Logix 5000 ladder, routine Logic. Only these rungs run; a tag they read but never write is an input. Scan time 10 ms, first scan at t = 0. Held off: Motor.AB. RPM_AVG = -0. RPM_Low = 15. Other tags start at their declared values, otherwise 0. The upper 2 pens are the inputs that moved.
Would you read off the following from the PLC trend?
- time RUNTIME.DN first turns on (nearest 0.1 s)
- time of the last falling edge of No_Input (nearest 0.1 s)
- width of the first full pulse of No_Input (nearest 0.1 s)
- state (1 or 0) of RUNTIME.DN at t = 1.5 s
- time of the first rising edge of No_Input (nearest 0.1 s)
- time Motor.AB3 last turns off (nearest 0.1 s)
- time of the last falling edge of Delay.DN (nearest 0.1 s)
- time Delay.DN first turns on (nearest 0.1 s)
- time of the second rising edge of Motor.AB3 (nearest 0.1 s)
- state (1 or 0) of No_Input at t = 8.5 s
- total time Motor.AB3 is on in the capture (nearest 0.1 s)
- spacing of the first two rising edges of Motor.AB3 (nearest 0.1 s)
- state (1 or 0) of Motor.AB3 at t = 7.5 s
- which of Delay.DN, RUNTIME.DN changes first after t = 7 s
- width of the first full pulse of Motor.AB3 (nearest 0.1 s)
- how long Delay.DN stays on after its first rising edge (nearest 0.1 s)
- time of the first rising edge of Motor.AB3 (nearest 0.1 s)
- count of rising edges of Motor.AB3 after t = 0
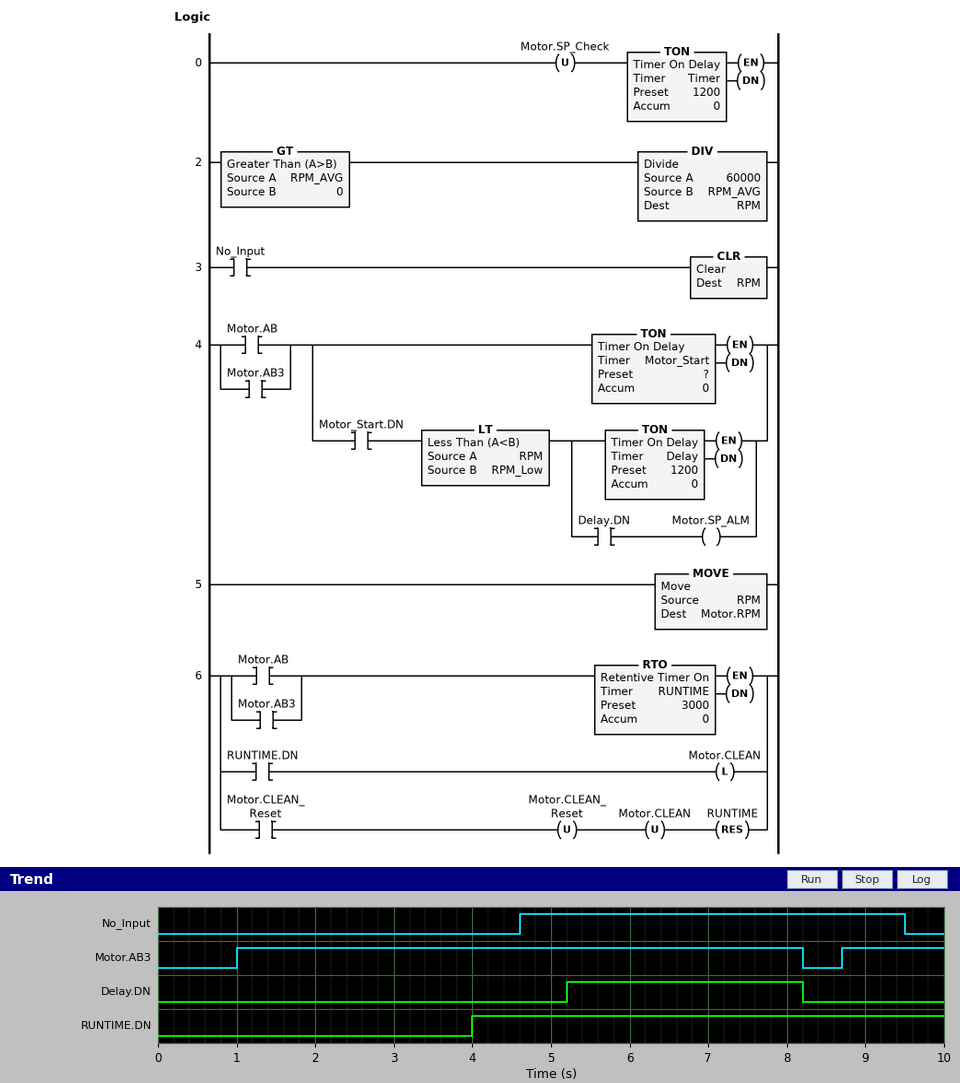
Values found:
4.0 s
9.5 s
4.9 s
0
4.6 s
8.2 s
8.2 s
5.2 s
8.7 s
1
8.5 s
7.7 s
1
Delay.DN
7.2 s
3.0 s
1.0 s
2
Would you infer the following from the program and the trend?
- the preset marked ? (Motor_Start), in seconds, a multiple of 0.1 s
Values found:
3.0 s
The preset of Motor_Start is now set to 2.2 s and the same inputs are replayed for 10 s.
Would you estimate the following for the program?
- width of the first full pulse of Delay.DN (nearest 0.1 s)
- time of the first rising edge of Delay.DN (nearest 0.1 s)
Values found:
3.8 s
4.4 s
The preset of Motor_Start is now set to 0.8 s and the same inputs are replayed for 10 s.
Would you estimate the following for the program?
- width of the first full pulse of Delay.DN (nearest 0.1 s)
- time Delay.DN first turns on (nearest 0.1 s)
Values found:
5.2 s
3.0 s
